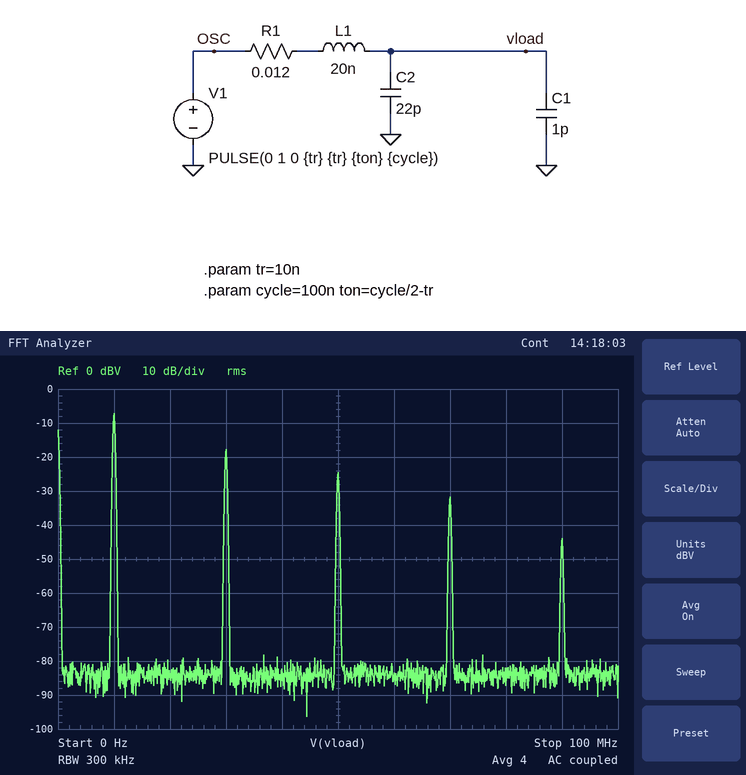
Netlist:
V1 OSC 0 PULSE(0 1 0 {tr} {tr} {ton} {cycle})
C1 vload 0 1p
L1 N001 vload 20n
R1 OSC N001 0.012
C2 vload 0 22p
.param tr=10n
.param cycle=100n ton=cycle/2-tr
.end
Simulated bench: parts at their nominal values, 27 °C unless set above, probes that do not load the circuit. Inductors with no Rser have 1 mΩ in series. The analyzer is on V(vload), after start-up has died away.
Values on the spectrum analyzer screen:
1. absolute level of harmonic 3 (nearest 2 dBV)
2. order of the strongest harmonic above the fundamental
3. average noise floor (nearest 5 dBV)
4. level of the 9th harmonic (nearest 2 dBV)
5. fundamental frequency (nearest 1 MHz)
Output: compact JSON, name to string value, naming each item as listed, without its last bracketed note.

{"absolute level of harmonic 3": "-18 dBV", "order of the strongest harmonic above the fundamental": "3", "average noise floor": "-85 dBV", "level of the 9th harmonic": "-44 dBV", "fundamental frequency": "10 MHz"}
